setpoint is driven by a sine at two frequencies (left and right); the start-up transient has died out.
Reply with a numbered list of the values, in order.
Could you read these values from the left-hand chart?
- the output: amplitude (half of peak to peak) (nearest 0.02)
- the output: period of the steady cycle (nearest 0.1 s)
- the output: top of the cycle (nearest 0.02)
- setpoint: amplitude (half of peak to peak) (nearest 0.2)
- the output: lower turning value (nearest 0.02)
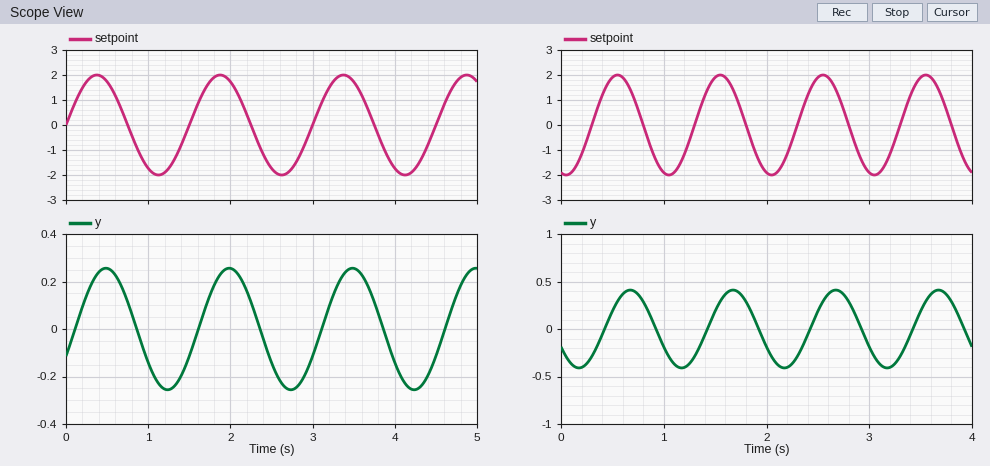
1. 0.26
2. 1.5 s
3. 0.26
4. 2.0
5. -0.26
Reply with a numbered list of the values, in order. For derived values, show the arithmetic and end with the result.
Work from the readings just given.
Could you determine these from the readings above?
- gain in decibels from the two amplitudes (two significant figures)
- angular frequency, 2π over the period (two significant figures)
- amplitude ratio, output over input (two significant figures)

1. 20 log10(0.26 / 2) = -18 dB
2. 2π / 1.5 = 4.2 rad/s
3. 0.26 / 2 = 0.13
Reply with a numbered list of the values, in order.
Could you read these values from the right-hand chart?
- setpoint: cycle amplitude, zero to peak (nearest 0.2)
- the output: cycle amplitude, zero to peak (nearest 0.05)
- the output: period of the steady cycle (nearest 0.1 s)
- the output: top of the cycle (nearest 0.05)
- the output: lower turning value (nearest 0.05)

1. 2.0
2. 0.40
3. 1.0 s
4. 0.40
5. -0.40
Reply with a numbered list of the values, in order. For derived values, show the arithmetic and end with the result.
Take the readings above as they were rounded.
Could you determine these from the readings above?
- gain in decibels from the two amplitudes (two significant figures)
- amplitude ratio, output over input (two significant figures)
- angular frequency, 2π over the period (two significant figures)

1. 20 log10(0.4 / 2) = -14 dB
2. 0.4 / 2 = 0.20
3. 2π / 1 = 6.3 rad/s
